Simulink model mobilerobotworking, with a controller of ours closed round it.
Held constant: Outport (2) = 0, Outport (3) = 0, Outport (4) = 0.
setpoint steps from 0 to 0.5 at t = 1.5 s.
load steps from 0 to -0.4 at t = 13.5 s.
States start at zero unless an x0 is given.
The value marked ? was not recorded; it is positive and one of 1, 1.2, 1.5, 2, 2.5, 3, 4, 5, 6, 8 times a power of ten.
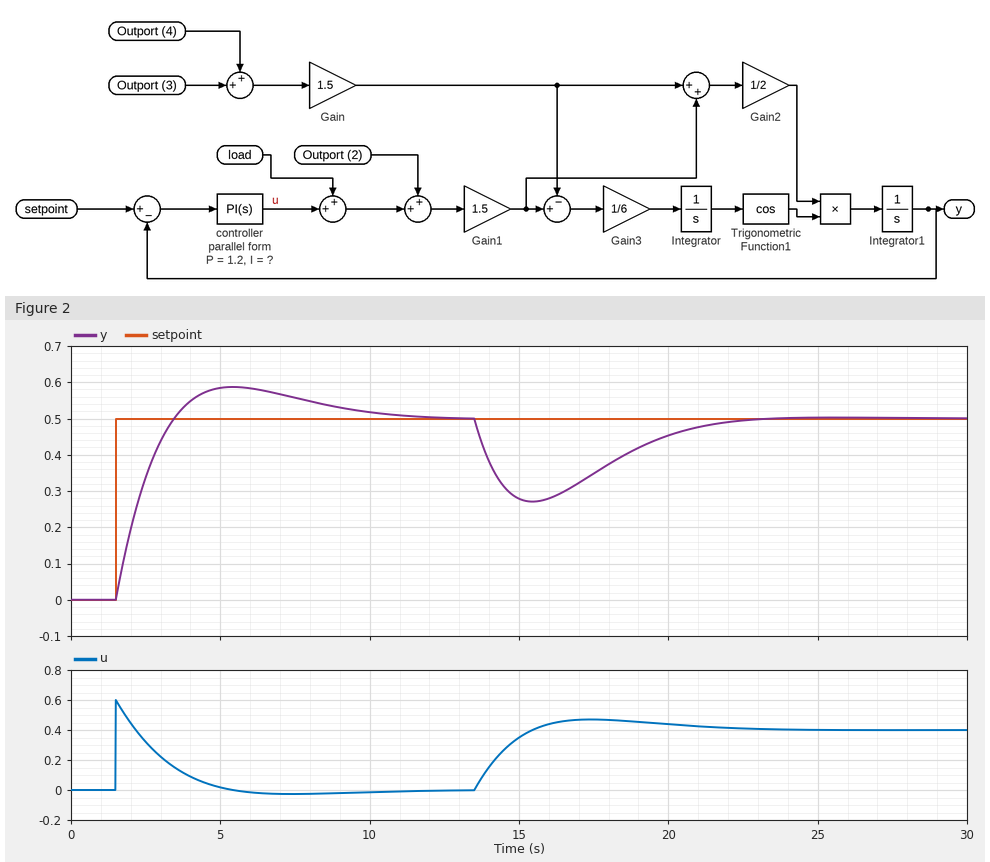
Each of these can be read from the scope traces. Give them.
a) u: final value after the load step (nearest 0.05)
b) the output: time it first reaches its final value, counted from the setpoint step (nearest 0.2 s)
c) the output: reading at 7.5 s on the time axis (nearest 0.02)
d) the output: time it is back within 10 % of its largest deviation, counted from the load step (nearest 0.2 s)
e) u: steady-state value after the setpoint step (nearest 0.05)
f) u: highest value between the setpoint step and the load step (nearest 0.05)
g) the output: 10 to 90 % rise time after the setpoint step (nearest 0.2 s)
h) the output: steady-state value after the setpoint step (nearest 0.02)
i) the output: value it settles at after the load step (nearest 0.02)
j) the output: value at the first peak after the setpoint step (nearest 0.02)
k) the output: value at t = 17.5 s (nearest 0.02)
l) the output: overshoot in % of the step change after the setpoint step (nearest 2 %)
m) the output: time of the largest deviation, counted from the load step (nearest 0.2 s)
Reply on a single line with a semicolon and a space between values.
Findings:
0.40; 2.0 s; 0.56; 7.6 s; 0.00; 0.60; 1.4 s; 0.50; 0.50; 0.58; 0.34; 18 %; 2.0 s
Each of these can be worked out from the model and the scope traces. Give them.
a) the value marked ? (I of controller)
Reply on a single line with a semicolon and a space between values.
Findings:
0.4
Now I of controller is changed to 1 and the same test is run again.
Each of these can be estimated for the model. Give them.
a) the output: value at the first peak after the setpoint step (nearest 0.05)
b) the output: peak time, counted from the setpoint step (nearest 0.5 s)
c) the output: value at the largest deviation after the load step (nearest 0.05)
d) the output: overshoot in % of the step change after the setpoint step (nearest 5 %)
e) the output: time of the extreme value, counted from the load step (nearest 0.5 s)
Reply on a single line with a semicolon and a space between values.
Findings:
0.65; 3.0 s; 0.30; 30 %; 1.5 s
